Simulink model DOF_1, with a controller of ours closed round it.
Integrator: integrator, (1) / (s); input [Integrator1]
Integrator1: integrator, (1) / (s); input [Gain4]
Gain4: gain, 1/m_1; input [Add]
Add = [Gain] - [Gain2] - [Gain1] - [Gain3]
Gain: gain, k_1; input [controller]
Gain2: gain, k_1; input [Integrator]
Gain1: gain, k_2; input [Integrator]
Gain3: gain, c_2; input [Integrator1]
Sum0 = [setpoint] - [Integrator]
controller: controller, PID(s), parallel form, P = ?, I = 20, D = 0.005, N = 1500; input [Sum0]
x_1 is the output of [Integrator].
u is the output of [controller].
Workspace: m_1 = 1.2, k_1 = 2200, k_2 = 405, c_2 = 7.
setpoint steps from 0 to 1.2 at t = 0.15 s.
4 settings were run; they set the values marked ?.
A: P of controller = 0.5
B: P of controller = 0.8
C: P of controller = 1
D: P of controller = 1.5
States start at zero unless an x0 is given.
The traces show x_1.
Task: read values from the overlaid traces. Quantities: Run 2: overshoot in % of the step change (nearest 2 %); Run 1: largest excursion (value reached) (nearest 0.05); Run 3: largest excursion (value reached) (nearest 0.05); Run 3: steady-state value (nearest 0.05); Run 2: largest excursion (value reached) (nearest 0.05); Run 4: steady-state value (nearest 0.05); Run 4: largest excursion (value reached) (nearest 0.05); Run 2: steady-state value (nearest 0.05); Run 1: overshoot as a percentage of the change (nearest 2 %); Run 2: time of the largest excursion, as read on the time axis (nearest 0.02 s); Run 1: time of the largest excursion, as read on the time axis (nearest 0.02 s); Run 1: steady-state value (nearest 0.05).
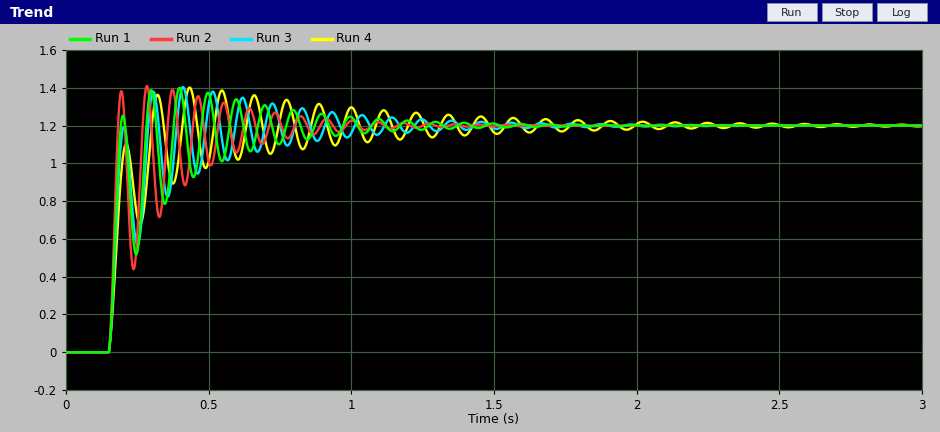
18 %
1.40
1.40
1.20
1.40
1.20
1.40
1.20
16 %
0.28 s
0.40 s
1.20
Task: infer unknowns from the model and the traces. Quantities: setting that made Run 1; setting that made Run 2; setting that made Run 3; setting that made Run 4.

C
D
B
A
